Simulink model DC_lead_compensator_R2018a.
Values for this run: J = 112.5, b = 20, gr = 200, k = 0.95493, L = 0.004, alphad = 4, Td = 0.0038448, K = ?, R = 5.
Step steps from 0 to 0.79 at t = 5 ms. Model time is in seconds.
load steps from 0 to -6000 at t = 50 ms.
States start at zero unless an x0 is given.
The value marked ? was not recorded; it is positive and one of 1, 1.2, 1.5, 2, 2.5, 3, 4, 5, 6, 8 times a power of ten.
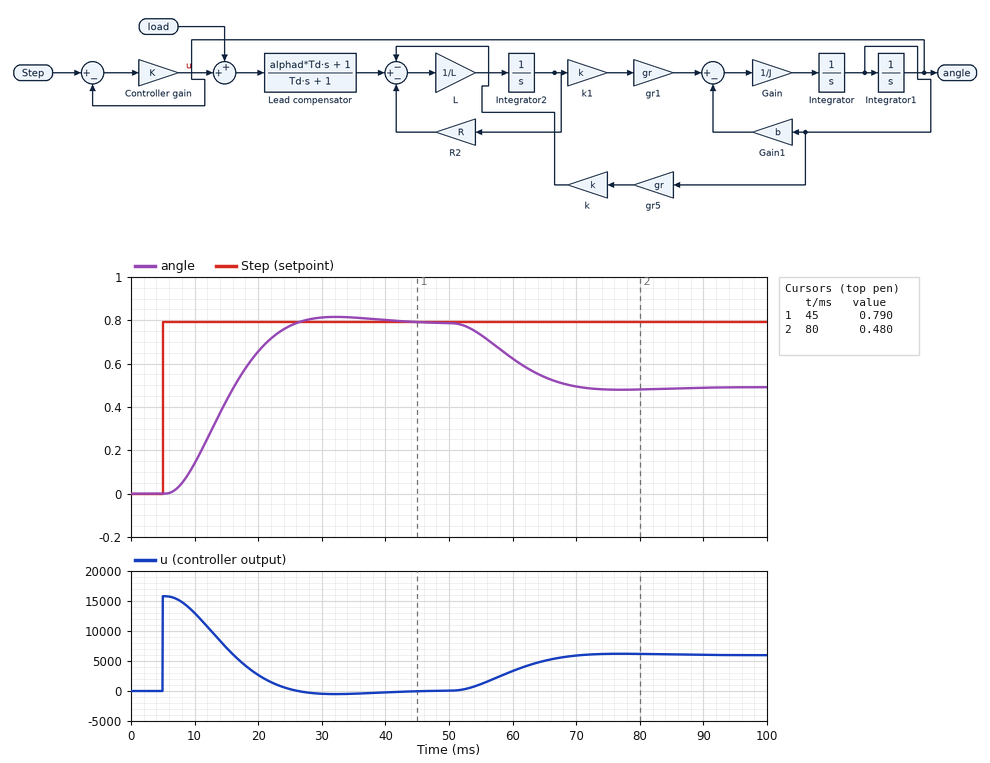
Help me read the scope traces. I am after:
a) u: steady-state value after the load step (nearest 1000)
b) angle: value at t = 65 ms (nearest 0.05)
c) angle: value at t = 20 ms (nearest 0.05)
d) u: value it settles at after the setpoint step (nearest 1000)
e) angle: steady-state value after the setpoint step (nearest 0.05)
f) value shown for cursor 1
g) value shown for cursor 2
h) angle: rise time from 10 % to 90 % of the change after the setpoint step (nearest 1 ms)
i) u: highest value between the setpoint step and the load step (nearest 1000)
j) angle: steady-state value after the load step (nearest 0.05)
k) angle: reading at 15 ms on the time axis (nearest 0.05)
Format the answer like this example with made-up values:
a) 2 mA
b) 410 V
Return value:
a) 6000
b) 0.55
c) 0.65
d) 0
e) 0.80
f) 0.790
g) 0.480
h) 13 ms
i) 16000
j) 0.50
k) 0.45
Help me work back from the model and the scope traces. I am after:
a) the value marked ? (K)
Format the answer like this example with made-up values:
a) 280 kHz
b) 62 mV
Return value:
a) 20000
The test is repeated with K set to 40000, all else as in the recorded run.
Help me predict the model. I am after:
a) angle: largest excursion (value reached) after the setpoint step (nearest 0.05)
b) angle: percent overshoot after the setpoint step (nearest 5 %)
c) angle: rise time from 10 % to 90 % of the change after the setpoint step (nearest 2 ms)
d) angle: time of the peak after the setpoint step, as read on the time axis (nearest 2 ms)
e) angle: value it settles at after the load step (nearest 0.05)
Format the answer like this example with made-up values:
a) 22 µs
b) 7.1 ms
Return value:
a) 0.95
b) 20 %
c) 6 ms
d) 20 ms
e) 0.65
